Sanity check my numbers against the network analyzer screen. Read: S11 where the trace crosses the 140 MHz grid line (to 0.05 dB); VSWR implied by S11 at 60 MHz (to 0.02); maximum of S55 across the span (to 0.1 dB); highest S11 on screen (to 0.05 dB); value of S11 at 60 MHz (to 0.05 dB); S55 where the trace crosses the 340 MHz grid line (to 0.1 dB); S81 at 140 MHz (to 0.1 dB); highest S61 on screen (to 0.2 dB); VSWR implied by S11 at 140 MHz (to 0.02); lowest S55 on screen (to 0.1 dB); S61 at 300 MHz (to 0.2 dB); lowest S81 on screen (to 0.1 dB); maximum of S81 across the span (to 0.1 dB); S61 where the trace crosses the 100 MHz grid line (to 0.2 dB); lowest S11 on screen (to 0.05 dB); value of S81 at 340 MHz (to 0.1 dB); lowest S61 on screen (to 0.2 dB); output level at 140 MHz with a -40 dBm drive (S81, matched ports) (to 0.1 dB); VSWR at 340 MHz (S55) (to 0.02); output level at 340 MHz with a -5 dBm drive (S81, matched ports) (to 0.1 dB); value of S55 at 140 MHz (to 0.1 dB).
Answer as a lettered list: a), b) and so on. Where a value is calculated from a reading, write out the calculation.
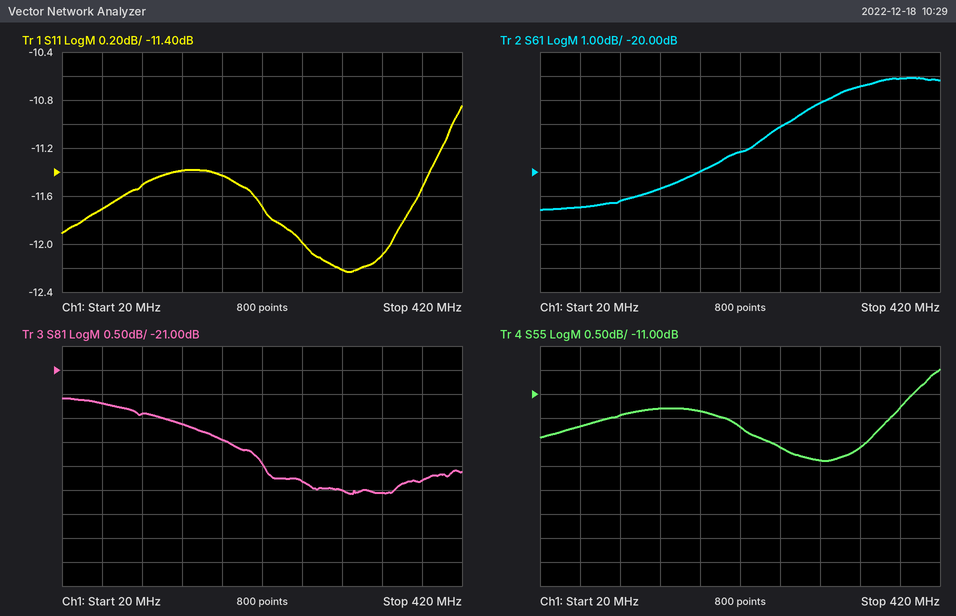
a) -11.40 dB
b) |Γ| = 10^(-11.7/20) = 0.2600; VSWR = (1 + 0.2600)/(1 − 0.2600) ≈ 1.70
c) -10.5 dB
d) -10.85 dB
e) -11.70 dB
f) -12.1 dB
g) -22.1 dB
h) -16.0 dB
i) |Γ| = 10^(-11.4/20) = 0.2692; VSWR = (1 + 0.2692)/(1 − 0.2692) ≈ 1.74
j) -12.4 dB
k) -17.2 dB
l) -23.6 dB
m) -21.6 dB
n) -21.2 dB
o) -12.25 dB
p) -23.6 dB
q) -21.6 dB
r) -40 dBm + (-22.1 dB) = -62.1 dBm
s) |Γ| = 10^(-12.1/20) = 0.2483; VSWR = (1 + 0.2483)/(1 − 0.2483) ≈ 1.66
t) -5 dBm + (-23.6 dB) = -28.6 dBm
u) -11.3 dB
